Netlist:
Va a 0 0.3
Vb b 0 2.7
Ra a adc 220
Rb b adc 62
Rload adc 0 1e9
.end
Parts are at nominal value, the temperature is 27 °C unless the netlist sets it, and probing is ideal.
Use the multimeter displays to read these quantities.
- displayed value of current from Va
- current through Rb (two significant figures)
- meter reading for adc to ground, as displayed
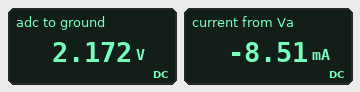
-8.51 mA
8.5 mA
2.172 V
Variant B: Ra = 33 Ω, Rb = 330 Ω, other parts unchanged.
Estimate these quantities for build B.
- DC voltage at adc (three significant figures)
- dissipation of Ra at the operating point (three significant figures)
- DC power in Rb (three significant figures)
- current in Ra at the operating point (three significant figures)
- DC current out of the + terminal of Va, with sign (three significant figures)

518 mV
1.44 mW
14.4 mW
6.61 mA
-6.61 mA
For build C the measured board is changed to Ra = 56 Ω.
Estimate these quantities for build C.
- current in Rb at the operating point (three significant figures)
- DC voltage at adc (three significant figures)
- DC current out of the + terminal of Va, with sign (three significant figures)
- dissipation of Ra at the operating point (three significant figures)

20.3 mA
1.44 V
-20.3 mA
23.2 mW
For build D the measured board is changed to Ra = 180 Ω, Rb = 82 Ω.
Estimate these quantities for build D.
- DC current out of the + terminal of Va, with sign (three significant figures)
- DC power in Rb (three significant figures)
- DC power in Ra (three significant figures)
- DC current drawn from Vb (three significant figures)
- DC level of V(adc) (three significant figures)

-9.16 mA
6.88 mW
15.1 mW
9.16 mA
1.95 V
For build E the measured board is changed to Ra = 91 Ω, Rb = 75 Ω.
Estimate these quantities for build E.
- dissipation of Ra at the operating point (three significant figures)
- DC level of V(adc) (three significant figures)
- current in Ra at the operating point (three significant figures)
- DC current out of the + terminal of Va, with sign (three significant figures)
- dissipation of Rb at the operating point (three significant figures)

19.0 mW
1.62 V
14.5 mA
-14.5 mA
15.7 mW
